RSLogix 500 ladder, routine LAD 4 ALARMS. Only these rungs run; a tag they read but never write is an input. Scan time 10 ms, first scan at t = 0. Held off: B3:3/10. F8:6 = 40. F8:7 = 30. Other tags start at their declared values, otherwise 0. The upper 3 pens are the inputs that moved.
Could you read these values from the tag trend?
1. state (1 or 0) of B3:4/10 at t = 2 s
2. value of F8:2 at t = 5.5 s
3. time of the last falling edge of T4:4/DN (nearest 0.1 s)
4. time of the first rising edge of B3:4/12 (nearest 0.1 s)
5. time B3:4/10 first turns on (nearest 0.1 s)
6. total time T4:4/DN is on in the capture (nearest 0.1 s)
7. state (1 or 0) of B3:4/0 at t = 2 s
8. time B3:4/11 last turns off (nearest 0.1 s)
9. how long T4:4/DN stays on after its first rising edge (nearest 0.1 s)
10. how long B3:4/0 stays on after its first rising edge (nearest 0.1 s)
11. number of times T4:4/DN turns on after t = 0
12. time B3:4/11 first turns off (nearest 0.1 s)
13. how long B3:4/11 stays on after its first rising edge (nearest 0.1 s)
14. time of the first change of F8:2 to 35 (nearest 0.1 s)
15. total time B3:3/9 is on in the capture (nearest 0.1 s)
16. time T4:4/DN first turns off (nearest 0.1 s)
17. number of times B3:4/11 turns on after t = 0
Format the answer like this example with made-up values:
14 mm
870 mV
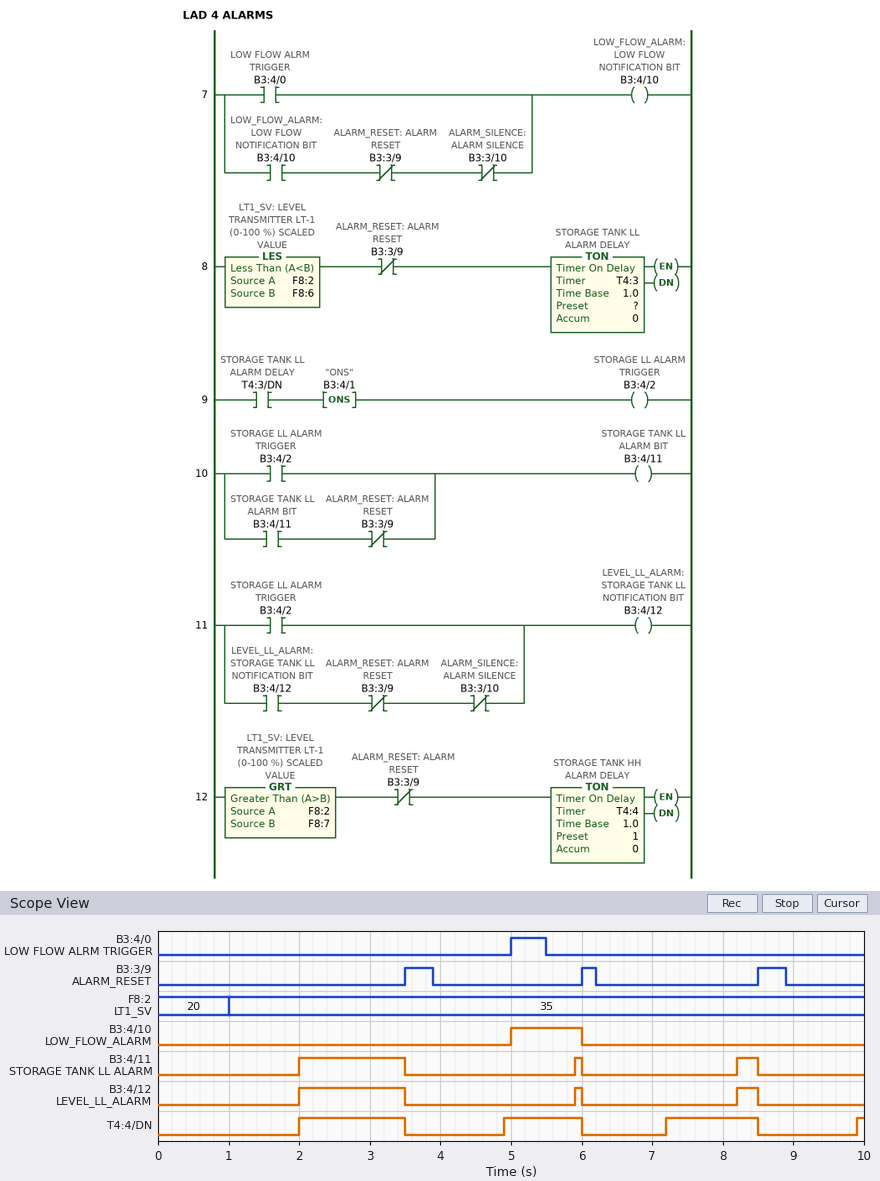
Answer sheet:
0
35
8.5 s
2.0 s
5.0 s
4.0 s
0
8.5 s
1.5 s
0.5 s
4
3.5 s
1.5 s
1.0 s
1.0 s
3.5 s
3
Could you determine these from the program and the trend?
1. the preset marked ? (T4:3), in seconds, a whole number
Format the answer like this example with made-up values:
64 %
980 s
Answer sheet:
2 s
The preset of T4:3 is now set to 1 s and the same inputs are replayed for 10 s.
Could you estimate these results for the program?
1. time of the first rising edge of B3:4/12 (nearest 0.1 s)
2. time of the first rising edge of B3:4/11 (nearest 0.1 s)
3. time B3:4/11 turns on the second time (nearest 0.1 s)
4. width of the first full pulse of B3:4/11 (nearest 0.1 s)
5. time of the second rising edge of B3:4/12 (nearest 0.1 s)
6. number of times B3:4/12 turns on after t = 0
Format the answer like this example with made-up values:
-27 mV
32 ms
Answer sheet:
1.0 s
1.0 s
4.9 s
2.5 s
4.9 s
4
